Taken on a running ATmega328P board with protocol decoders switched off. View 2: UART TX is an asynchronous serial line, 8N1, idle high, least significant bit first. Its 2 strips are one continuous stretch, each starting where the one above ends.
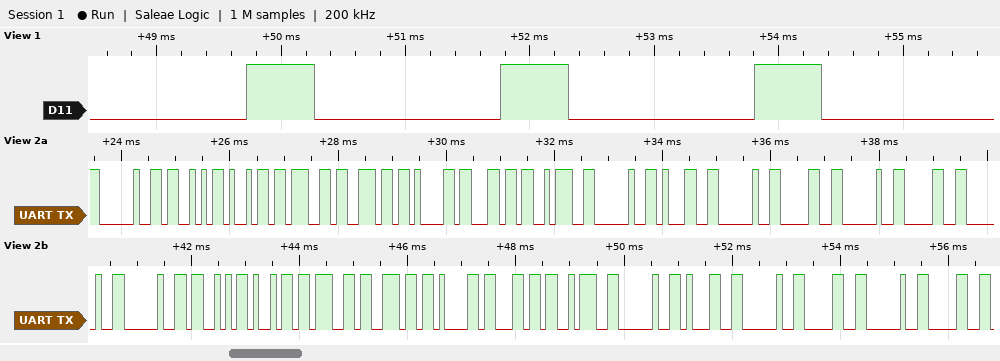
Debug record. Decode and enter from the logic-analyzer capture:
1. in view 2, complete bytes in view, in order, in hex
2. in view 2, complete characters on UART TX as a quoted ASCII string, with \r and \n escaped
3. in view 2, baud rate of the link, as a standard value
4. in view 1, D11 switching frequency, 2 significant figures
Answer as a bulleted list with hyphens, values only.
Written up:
- 0x20 0x53 0x69 0x67 0x6E 0x61 0x6C 0x3A 0x20 0x31 0x20 0x30 0x20 0x30 0x20 0x20 0x53 0x69 0x67 0x6E 0x61 0x6C 0x3A 0x20 0x31 0x20 0x30 0x20 0x30
- " Signal: 1 0 0  Signal: 1 0 0"
- 9600 baud
- 490 Hz
